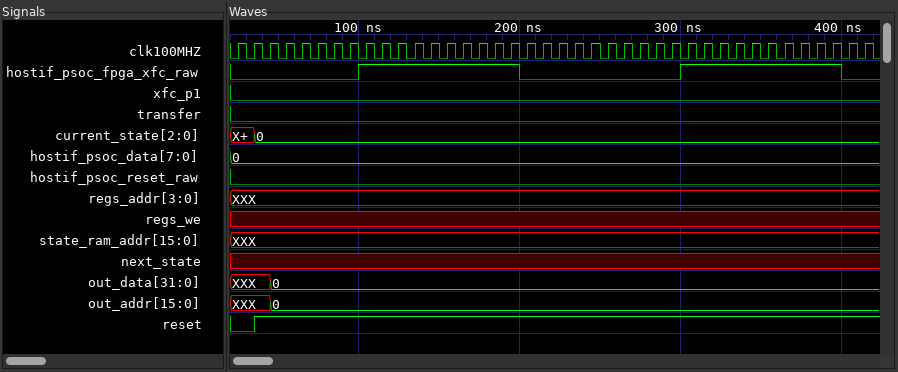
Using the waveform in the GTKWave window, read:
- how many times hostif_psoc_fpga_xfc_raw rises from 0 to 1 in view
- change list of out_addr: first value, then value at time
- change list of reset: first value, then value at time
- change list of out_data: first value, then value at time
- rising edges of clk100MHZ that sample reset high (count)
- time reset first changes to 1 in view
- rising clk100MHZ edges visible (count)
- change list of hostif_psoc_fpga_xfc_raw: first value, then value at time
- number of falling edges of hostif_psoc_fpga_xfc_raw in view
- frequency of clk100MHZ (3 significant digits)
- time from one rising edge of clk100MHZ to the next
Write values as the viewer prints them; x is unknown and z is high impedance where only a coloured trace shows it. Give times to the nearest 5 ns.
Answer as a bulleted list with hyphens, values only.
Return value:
- 2
- XXX, 0 at 45 ns
- 0, 1 at 35 ns
- XXX, 0 at 45 ns
- 38
- 35 ns
- 40
- 0, 1 at 100 ns, 0 at 200 ns, 1 at 300 ns, 0 at 400 ns
- 2
- 100 MHz
- 10 ns
